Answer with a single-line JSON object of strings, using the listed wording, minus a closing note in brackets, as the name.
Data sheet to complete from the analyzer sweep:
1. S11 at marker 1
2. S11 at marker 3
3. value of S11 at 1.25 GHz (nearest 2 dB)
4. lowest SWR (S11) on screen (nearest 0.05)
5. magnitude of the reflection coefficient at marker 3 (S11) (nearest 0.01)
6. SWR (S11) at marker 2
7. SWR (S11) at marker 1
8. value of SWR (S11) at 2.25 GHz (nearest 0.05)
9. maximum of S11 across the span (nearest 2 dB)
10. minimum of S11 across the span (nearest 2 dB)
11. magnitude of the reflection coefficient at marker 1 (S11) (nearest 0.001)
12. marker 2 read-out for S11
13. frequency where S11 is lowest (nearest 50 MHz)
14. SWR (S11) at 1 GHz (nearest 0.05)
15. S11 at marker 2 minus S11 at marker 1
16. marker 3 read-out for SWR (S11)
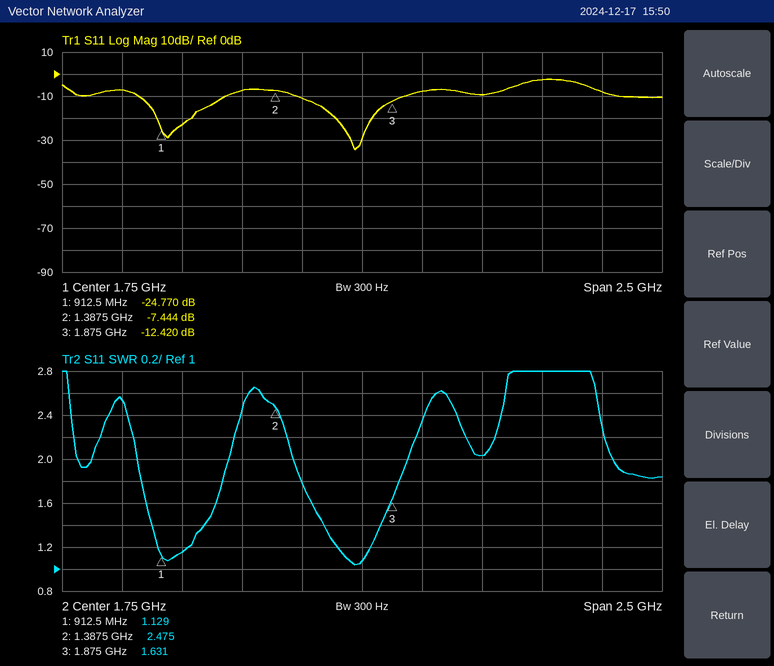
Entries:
{"S11 at marker 1": "-24.770 dB", "S11 at marker 3": "-12.420 dB", "value of S11 at 1.25 GHz": "-8 dB", "lowest SWR (S11) on screen": "1.05", "magnitude of the reflection coefficient at marker 3 (S11)": "0.24", "SWR (S11) at marker 2": "2.475", "SWR (S11) at marker 1": "1.129", "value of SWR (S11) at 2.25 GHz": "2.05", "maximum of S11 across the span": "-2 dB", "minimum of S11 across the span": "-34 dB", "magnitude of the reflection coefficient at marker 1 (S11)": "0.058", "marker 2 read-out for S11": "-7.444 dB", "frequency where S11 is lowest": "1.70 GHz", "SWR (S11) at 1 GHz": "1.15", "S11 at marker 2 minus S11 at marker 1": "17.326 dB", "marker 3 read-out for SWR": "1.631"}
